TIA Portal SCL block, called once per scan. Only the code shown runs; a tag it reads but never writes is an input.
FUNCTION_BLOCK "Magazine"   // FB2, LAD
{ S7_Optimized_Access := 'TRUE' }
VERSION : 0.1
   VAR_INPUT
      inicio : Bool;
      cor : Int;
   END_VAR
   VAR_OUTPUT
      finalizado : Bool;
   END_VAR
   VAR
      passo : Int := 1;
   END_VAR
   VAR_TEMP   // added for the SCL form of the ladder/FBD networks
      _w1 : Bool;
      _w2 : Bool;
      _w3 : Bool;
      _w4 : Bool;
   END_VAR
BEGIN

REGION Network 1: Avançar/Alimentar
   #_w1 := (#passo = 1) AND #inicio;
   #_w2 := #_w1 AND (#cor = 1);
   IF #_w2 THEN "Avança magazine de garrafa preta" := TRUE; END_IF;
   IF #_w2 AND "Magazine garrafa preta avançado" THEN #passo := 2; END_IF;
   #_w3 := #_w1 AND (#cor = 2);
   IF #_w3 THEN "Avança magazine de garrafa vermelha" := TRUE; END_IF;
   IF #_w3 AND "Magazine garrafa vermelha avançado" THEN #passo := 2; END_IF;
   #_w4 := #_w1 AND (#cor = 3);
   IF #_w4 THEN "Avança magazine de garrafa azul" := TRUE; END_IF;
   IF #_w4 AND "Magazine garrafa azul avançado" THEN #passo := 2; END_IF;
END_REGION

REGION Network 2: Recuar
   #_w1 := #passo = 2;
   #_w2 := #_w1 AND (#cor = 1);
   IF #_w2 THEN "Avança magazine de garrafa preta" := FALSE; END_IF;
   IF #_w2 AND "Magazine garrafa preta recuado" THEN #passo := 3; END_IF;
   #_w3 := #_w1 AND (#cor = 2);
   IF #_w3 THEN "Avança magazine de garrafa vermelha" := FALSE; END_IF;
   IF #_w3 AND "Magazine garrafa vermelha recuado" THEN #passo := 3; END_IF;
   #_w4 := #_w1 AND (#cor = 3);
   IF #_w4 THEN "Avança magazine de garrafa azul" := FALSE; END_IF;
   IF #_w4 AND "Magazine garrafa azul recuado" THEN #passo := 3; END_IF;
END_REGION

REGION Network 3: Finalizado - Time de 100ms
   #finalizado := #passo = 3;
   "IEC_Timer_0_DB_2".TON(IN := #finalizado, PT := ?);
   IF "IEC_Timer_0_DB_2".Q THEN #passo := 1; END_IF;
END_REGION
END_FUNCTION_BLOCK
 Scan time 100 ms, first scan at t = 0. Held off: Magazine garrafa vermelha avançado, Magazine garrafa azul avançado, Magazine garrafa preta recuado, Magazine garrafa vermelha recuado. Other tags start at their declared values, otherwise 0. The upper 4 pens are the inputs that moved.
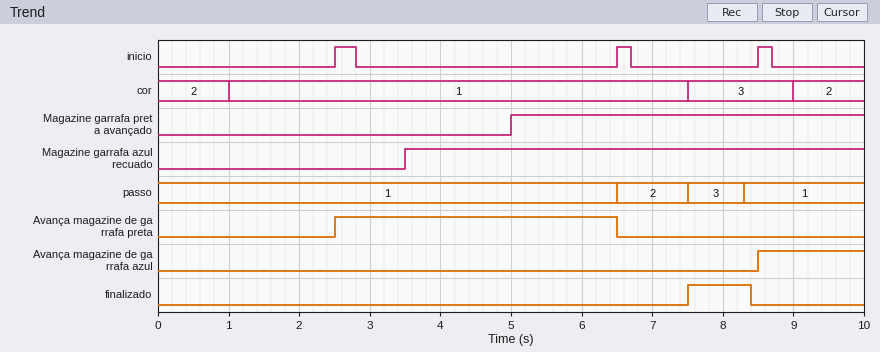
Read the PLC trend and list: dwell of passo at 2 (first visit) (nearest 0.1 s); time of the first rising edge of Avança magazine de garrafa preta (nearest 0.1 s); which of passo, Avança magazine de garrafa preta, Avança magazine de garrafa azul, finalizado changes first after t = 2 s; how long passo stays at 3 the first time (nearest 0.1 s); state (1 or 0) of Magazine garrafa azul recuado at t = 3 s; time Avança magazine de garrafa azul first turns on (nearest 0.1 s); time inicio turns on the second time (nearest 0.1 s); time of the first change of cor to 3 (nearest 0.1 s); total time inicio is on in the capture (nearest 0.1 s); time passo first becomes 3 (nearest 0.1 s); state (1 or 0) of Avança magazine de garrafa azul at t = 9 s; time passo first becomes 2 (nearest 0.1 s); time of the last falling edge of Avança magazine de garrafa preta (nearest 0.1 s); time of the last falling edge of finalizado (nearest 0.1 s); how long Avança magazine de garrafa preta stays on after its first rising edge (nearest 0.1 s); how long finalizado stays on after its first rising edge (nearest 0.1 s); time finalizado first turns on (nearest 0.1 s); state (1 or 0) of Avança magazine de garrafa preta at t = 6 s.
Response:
1.0 s
2.5 s
Avança magazine de garrafa preta
0.8 s
0
8.5 s
6.5 s
7.5 s
0.7 s
7.5 s
1
6.5 s
6.5 s
8.4 s
4.0 s
0.9 s
7.5 s
1
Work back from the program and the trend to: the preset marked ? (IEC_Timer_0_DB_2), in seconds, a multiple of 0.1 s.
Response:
0.8 s
